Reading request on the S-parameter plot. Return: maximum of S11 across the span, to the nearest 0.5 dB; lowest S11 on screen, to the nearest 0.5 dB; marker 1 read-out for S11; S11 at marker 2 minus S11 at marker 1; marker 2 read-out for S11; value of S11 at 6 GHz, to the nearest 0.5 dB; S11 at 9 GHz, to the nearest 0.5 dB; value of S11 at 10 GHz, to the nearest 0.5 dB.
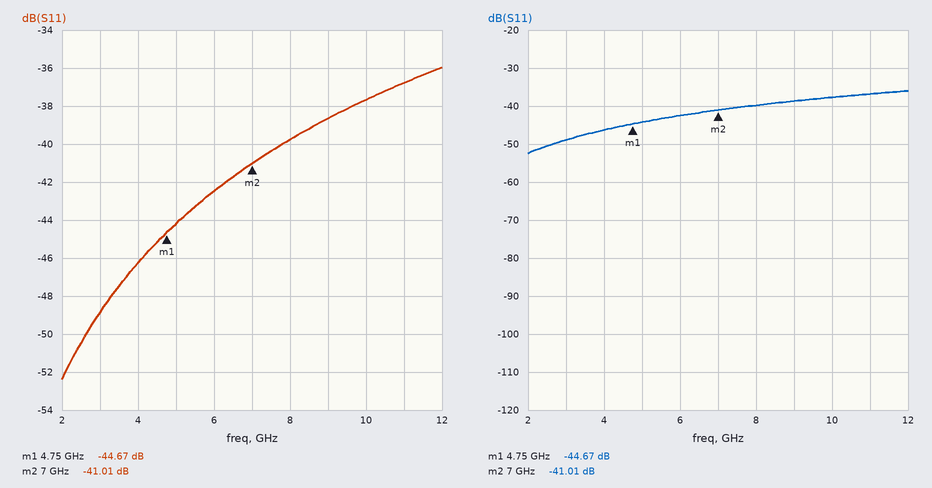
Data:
-36.0 dB
-52.5 dB
-44.67 dB
3.66 dB
-41.01 dB
-42.5 dB
-38.5 dB
-37.5 dB
